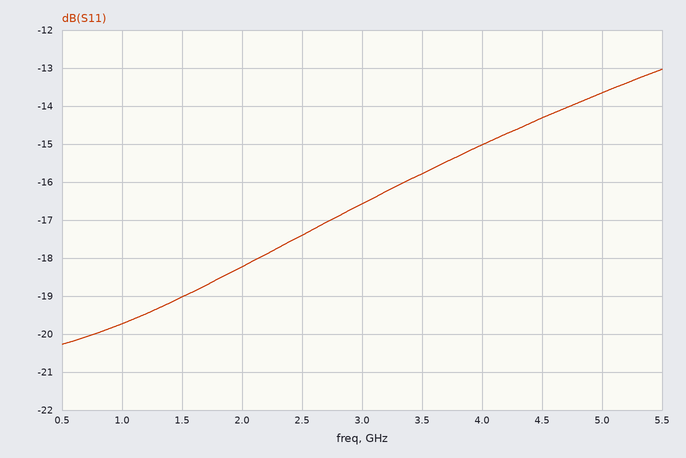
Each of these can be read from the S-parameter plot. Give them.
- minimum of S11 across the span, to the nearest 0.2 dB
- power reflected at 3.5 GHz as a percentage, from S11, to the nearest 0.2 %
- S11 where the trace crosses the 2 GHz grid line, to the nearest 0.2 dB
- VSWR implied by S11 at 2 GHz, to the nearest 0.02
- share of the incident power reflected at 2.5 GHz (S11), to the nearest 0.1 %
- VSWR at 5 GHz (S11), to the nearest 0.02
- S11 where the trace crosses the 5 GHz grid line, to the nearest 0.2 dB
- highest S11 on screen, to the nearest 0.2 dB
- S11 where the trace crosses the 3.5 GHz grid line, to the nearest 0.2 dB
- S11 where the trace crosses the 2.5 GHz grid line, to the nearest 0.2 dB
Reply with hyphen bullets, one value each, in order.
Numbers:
- -20.2 dB
- 2.6 %
- -18.2 dB
- 1.28
- 1.8 %
- 1.52
- -13.6 dB
- -13.0 dB
- -15.8 dB
- -17.4 dB
